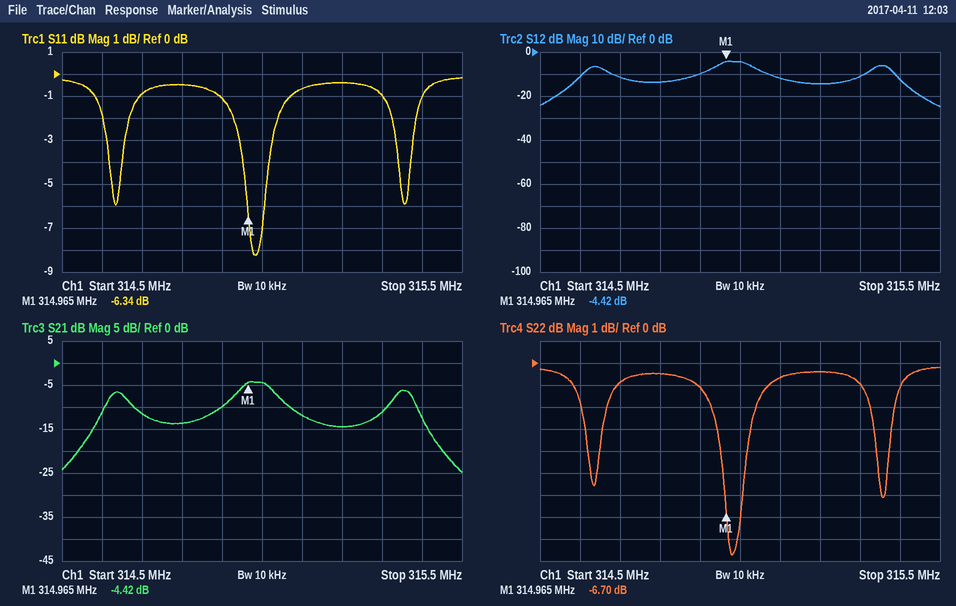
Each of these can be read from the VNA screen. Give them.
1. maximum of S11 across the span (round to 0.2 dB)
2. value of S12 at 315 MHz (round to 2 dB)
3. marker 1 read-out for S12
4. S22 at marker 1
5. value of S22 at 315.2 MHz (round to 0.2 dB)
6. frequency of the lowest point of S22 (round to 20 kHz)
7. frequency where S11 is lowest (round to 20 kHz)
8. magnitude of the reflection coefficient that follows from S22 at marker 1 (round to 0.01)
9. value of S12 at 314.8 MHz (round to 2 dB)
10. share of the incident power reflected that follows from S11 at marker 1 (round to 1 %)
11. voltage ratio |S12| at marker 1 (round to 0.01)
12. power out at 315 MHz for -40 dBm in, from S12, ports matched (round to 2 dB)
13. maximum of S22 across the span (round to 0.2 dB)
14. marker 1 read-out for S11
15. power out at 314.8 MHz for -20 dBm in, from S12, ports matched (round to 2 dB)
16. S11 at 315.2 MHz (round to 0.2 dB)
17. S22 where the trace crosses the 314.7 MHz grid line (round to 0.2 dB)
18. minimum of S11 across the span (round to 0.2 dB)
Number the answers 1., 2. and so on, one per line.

1. -0.2 dB
2. -4 dB
3. -4.42 dB
4. -6.70 dB
5. -0.4 dB
6. 314.98 MHz
7. 314.98 MHz
8. 0.46
9. -14 dB
10. 23 %
11. 0.60
12. -44 dBm
13. -0.2 dB
14. -6.34 dB
15. -34 dBm
16. -0.4 dB
17. -0.8 dB
18. -8.2 dB
